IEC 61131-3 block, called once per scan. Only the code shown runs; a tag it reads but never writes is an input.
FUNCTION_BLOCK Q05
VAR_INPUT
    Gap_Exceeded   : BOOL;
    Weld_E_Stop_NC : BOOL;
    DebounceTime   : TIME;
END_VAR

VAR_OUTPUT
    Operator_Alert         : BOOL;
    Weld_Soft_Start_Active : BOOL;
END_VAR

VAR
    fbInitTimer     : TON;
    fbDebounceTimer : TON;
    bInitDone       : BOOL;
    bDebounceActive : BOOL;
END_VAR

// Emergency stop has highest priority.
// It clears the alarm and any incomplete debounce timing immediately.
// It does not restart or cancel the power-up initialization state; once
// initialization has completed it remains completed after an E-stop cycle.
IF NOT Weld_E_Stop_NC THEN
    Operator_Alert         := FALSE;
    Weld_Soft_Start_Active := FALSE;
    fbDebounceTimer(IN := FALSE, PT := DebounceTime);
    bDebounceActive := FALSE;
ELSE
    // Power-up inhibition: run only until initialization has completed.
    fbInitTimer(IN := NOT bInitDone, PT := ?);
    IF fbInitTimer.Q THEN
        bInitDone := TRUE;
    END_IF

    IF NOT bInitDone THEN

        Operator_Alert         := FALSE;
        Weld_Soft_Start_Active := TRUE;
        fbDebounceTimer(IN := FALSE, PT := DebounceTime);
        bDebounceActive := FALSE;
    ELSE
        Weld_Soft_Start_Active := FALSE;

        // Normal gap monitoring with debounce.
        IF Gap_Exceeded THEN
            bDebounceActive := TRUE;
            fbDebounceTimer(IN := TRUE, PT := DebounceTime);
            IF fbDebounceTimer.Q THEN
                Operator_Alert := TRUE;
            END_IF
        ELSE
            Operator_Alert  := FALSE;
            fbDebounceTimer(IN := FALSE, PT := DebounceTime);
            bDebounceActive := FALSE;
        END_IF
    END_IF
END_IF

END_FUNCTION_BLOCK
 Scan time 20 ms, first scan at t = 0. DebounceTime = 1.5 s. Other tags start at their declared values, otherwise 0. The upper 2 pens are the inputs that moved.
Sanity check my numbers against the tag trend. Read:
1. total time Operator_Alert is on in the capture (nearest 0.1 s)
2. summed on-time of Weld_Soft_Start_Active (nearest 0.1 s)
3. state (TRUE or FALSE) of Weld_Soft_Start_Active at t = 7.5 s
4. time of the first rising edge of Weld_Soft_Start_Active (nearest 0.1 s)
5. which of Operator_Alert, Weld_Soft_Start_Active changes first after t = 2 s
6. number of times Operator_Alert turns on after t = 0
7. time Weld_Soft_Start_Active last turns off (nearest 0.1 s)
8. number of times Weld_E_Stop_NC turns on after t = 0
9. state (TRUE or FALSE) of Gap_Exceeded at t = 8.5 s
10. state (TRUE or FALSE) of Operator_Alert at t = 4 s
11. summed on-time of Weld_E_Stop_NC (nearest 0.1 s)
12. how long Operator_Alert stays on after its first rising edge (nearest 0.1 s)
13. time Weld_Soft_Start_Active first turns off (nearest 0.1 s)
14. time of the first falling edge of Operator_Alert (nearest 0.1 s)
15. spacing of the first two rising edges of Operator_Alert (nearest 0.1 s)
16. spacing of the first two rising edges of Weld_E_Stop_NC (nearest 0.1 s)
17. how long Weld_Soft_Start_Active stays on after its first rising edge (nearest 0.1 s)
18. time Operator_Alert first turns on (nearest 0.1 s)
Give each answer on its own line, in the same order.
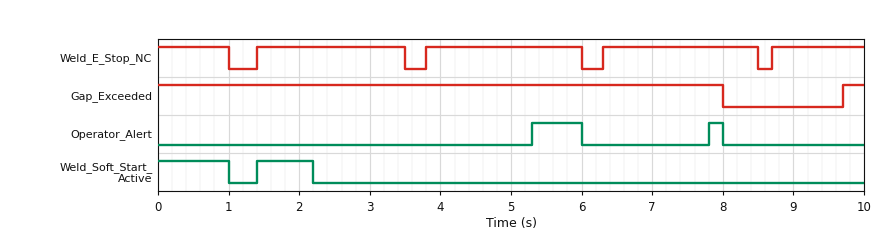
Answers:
0.9 s
1.8 s
FALSE
1.4 s
Weld_Soft_Start_Active
2
2.2 s
4
FALSE
FALSE
8.8 s
0.7 s
1.0 s
6.0 s
2.5 s
2.4 s
0.8 s
5.3 s
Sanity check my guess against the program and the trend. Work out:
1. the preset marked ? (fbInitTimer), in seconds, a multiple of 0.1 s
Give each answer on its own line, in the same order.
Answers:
2.2 s
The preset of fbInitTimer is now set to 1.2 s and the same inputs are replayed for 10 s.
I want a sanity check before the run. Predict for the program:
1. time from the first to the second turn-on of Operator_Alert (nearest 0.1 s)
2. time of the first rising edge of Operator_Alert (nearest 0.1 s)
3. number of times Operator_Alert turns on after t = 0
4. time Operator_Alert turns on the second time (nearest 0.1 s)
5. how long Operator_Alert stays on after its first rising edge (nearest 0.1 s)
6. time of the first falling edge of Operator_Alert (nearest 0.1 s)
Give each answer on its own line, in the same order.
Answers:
2.4 s
2.9 s
3
5.3 s
0.6 s
3.5 s
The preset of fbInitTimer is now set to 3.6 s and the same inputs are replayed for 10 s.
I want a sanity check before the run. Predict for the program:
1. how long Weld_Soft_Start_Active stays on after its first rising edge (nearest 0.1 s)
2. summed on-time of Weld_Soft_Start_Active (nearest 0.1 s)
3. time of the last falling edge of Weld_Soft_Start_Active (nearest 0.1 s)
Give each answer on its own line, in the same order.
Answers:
2.1 s
3.1 s
3.5 s
